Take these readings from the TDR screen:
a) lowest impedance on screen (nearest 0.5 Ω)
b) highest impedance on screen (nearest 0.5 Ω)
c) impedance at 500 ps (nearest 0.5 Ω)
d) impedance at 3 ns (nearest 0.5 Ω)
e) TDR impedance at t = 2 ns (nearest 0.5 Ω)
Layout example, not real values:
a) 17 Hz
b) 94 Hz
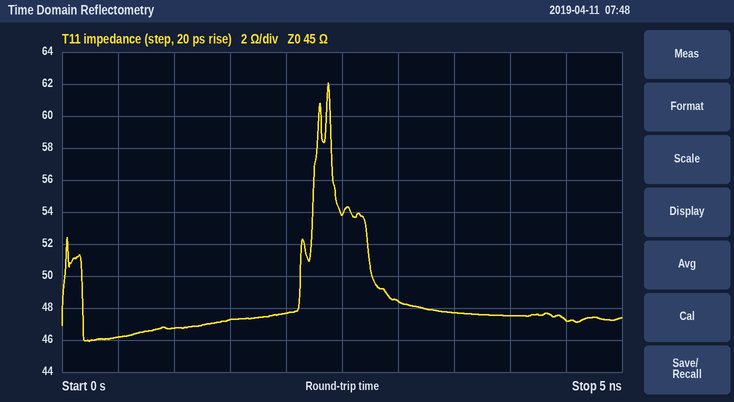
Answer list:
a) 46.0 Ω
b) 62.0 Ω
c) 46.0 Ω
d) 48.5 Ω
e) 47.5 Ω
